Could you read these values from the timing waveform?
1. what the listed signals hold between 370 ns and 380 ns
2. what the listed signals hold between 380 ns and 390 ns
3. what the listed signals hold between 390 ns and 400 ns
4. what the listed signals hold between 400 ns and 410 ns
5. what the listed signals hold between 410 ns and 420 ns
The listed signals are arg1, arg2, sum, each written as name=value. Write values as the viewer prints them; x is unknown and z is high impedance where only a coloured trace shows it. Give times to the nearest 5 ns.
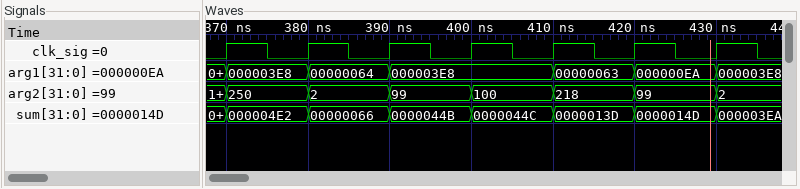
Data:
arg1=000003E8, arg2=250, sum=000004E2
arg1=00000064, arg2=2, sum=00000066
arg1=000003E8, arg2=99, sum=0000044B
arg1=000003E8, arg2=100, sum=0000044C
arg1=00000063, arg2=218, sum=0000013D
